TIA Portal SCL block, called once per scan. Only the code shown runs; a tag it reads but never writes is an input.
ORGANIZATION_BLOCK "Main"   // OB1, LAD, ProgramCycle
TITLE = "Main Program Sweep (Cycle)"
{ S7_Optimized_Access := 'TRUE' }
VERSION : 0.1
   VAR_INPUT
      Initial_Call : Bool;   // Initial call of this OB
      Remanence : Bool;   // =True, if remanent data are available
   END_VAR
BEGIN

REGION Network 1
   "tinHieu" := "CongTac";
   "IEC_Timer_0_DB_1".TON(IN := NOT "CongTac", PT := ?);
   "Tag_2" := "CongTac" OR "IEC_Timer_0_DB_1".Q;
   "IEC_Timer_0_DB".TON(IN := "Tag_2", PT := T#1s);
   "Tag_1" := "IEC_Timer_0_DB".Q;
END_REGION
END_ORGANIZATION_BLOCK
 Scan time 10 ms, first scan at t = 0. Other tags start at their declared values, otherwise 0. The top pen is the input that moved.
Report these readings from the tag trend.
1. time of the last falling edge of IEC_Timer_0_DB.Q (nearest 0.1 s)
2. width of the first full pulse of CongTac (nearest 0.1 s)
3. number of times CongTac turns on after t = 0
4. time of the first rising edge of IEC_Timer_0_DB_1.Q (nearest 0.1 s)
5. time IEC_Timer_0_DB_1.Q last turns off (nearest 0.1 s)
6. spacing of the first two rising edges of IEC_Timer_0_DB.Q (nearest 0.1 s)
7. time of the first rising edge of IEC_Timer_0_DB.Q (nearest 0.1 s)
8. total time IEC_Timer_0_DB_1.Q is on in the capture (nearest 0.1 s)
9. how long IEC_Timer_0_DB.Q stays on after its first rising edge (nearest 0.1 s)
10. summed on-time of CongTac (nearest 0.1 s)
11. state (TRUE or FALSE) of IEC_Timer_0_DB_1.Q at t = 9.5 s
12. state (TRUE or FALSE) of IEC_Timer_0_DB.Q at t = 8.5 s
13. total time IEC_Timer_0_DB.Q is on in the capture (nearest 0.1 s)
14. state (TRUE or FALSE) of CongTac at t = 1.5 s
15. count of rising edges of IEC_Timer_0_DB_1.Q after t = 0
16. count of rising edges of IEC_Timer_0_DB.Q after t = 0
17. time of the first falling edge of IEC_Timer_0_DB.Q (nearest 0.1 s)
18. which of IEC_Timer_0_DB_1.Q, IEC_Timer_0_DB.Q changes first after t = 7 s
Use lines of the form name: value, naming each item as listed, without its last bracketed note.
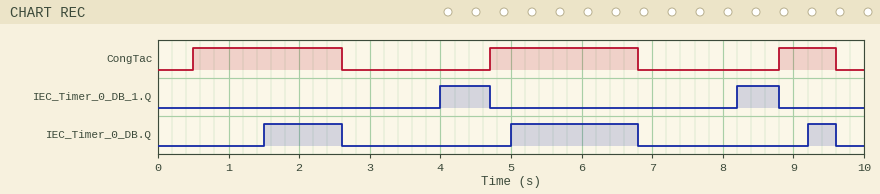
time of the last falling edge of IEC_Timer_0_DB.Q: 9.6 s
width of the first full pulse of CongTac: 2.1 s
number of times CongTac turns on after t = 0: 3
time of the first rising edge of IEC_Timer_0_DB_1.Q: 4.0 s
time IEC_Timer_0_DB_1.Q last turns off: 8.8 s
spacing of the first two rising edges of IEC_Timer_0_DB.Q: 3.5 s
time of the first rising edge of IEC_Timer_0_DB.Q: 1.5 s
total time IEC_Timer_0_DB_1.Q is on in the capture: 1.3 s
how long IEC_Timer_0_DB.Q stays on after its first rising edge: 1.1 s
summed on-time of CongTac: 5.0 s
state (TRUE or FALSE) of IEC_Timer_0_DB_1.Q at t = 9.5 s: FALSE
state (TRUE or FALSE) of IEC_Timer_0_DB.Q at t = 8.5 s: FALSE
total time IEC_Timer_0_DB.Q is on in the capture: 3.3 s
state (TRUE or FALSE) of CongTac at t = 1.5 s: TRUE
count of rising edges of IEC_Timer_0_DB_1.Q after t = 0: 2
count of rising edges of IEC_Timer_0_DB.Q after t = 0: 3
time of the first falling edge of IEC_Timer_0_DB.Q: 2.6 s
which of IEC_Timer_0_DB_1.Q, IEC_Timer_0_DB.Q changes first after t = 7 s: IEC_Timer_0_DB_1.Q
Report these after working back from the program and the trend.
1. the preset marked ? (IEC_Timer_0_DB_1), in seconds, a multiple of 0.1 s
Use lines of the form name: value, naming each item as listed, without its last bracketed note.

the preset marked ? (IEC_Timer_0_DB_1), in seconds, a multiple of 0.1 s: 1.4 s
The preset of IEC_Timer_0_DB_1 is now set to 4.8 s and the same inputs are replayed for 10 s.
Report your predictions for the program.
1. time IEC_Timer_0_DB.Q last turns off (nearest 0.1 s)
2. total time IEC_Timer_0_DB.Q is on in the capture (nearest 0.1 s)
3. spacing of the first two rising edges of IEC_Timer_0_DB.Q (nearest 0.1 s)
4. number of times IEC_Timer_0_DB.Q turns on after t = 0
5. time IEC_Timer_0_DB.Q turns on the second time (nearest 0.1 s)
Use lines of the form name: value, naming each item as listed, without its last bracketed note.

time IEC_Timer_0_DB.Q last turns off: 6.8 s
total time IEC_Timer_0_DB.Q is on in the capture: 2.2 s
spacing of the first two rising edges of IEC_Timer_0_DB.Q: 4.2 s
number of times IEC_Timer_0_DB.Q turns on after t = 0: 2
time IEC_Timer_0_DB.Q turns on the second time: 5.7 s
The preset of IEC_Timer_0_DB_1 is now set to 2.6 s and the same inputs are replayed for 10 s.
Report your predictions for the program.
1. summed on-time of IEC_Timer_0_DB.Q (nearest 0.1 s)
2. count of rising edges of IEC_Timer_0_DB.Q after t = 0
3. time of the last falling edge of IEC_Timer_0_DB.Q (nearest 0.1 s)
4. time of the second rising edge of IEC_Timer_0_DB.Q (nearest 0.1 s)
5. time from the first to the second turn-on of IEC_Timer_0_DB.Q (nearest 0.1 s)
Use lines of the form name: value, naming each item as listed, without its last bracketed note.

summed on-time of IEC_Timer_0_DB.Q: 2.2 s
count of rising edges of IEC_Timer_0_DB.Q after t = 0: 2
time of the last falling edge of IEC_Timer_0_DB.Q: 6.8 s
time of the second rising edge of IEC_Timer_0_DB.Q: 5.7 s
time from the first to the second turn-on of IEC_Timer_0_DB.Q: 4.2 s
